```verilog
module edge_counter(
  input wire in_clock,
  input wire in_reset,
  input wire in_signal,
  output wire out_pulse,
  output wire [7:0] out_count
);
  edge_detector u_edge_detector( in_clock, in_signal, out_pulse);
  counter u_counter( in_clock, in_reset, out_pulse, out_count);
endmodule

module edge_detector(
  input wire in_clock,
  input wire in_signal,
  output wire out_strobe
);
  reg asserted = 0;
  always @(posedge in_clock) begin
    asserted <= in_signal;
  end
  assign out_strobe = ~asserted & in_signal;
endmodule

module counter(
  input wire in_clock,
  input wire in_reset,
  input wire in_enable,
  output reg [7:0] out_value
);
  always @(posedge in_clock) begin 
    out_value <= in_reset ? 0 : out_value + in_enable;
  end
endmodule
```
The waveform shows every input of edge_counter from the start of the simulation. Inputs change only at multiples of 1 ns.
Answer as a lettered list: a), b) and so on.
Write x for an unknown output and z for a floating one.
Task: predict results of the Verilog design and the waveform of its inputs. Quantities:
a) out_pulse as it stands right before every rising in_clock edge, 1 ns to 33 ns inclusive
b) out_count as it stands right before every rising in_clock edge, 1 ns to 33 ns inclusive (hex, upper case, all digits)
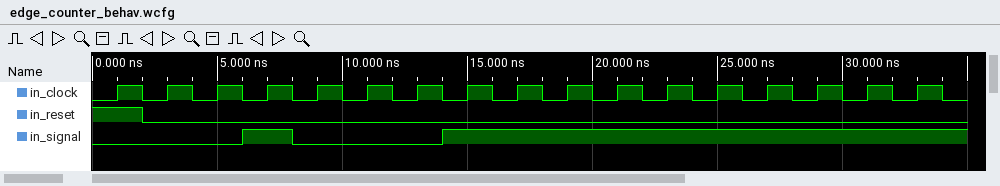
a) 0 0 0 1 0 0 0 1 0 0 0 0 0 0 0 0 0
b) x, 00, 00, 00, 01, 01, 01, 01, 02, 02, 02, 02, 02, 02, 02, 02, 02
